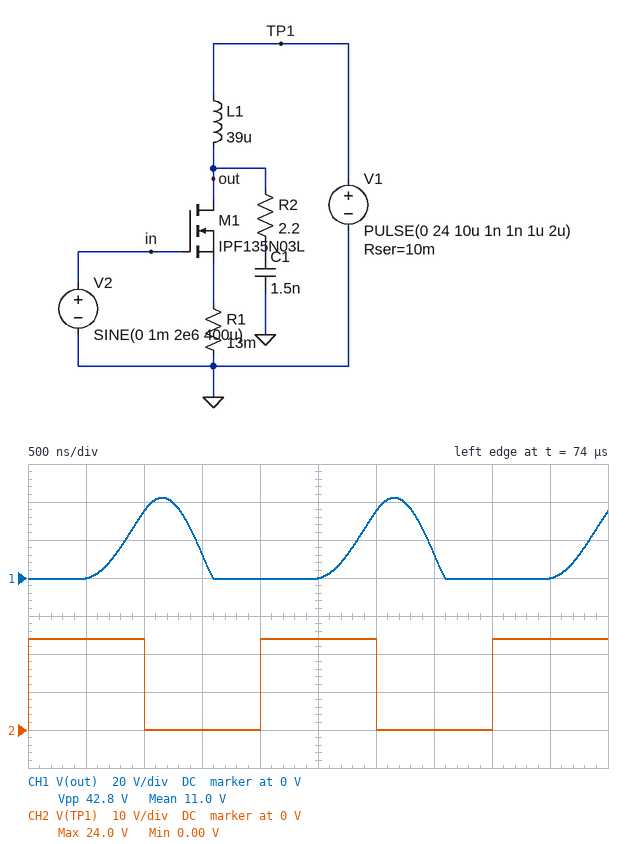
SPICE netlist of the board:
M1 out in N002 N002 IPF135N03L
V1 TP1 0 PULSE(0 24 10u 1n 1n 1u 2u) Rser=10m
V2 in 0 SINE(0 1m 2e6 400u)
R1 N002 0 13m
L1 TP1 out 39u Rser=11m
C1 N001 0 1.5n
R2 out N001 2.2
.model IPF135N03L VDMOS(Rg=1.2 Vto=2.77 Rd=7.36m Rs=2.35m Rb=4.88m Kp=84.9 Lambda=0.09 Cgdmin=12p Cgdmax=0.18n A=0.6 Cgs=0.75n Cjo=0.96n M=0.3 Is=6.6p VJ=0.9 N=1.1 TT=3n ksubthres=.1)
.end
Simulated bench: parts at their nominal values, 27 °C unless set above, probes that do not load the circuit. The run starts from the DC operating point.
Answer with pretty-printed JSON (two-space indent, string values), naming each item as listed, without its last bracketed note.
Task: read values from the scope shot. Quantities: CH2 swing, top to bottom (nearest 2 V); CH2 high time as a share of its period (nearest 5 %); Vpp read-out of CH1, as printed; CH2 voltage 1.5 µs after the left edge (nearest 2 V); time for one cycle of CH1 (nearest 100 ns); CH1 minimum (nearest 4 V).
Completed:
{
  "CH2 swing, top to bottom": "24 V",
  "CH2 high time as a share of its period": "50 %",
  "Vpp read-out of CH1, as printed": "42.8 V",
  "CH2 voltage 1.5 µs after the left edge": "0 V",
  "time for one cycle of CH1": "2.0 µs",
  "CH1 minimum": "0 V"
}
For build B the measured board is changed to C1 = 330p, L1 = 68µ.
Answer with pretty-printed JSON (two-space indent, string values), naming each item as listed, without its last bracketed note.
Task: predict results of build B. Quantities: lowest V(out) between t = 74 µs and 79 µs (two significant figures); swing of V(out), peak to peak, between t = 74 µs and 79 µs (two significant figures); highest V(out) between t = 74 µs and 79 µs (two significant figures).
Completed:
{
  "lowest V(out) between t = 74 µs and 79 µs": "-680 mV",
  "swing of V(out), peak to peak, between t = 74 µs and 79 µs": "52 V",
  "highest V(out) between t = 74 µs and 79 µs": "51 V"
}
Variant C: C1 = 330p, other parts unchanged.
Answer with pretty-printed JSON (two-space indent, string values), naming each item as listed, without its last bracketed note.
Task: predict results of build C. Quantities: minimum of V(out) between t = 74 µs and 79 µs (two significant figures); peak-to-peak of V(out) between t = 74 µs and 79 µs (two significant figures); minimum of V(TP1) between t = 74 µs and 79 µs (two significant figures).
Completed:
{
  "minimum of V(out) between t = 74 µs and 79 µs": "-690 mV",
  "peak-to-peak of V(out) between t = 74 µs and 79 µs": "54 V",
  "minimum of V(TP1) between t = 74 µs and 79 µs": "1.2 mV"
}
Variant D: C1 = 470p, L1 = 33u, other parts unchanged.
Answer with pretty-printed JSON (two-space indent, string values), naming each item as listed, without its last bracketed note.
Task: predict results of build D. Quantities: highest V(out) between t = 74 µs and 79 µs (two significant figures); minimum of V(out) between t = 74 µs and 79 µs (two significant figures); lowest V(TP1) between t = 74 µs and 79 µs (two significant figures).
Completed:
{
  "highest V(out) between t = 74 µs and 79 µs": "53 V",
  "minimum of V(out) between t = 74 µs and 79 µs": "-690 mV",
  "lowest V(TP1) between t = 74 µs and 79 µs": "1.3 mV"
}
